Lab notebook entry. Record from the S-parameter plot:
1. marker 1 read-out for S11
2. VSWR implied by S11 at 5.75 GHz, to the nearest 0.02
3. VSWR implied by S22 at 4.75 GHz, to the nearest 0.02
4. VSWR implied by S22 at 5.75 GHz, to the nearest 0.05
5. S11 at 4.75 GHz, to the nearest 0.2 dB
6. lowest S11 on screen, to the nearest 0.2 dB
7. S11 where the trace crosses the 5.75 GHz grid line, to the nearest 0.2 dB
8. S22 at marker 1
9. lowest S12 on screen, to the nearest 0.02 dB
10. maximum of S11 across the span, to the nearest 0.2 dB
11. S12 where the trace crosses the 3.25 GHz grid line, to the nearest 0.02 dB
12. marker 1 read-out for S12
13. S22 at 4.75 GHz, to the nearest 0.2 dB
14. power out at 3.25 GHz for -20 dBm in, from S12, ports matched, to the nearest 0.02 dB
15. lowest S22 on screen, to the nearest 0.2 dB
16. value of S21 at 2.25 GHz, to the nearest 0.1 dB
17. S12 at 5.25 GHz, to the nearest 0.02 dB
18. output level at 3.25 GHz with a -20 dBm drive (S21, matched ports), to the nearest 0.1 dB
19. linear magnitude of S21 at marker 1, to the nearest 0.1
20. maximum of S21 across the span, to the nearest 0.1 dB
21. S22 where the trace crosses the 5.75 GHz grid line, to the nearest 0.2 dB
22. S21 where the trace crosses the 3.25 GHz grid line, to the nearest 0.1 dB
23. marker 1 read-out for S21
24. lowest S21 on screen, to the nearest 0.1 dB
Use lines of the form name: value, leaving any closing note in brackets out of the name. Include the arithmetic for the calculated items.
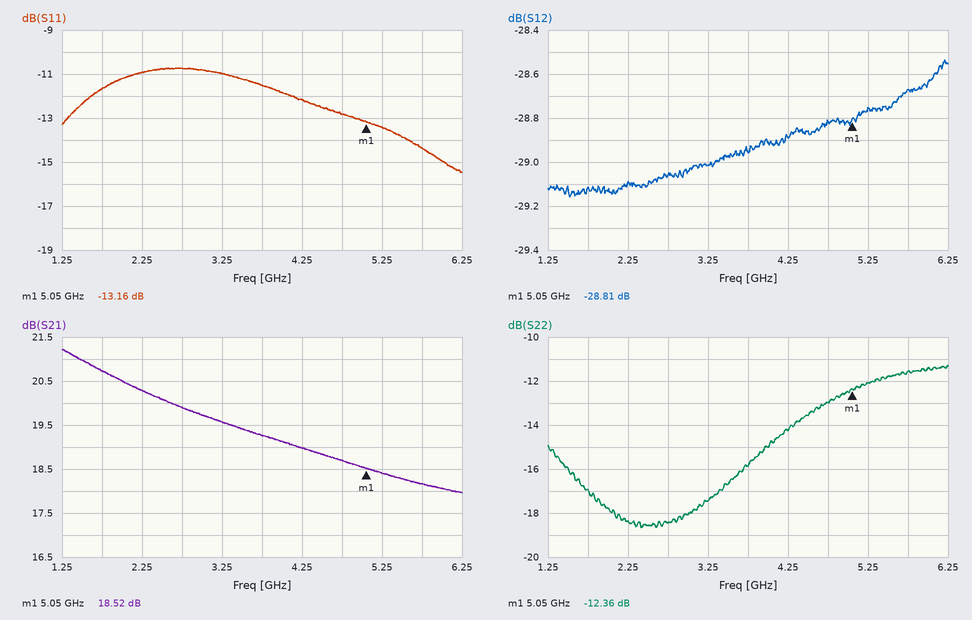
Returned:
marker 1 read-out for S11: -13.16 dB
VSWR implied by S11 at 5.75 GHz, to the nearest 0.02: |Γ| = 10^(-14.4/20) = 0.1905; VSWR = (1 + 0.1905)/(1 − 0.1905) ≈ 1.47, so 1.48 to the nearest 0.02
VSWR implied by S22 at 4.75 GHz, to the nearest 0.02: |Γ| = 10^(-13/20) = 0.2239; VSWR = (1 + 0.2239)/(1 − 0.2239) ≈ 1.58
VSWR implied by S22 at 5.75 GHz, to the nearest 0.05: |Γ| = 10^(-11.6/20) = 0.2630; VSWR = (1 + 0.2630)/(1 − 0.2630) ≈ 1.71, so 1.70 to the nearest 0.05
S11 at 4.75 GHz, to the nearest 0.2 dB: -12.8 dB
lowest S11 on screen, to the nearest 0.2 dB: -15.4 dB
S11 where the trace crosses the 5.75 GHz grid line, to the nearest 0.2 dB: -14.4 dB
S22 at marker 1: -12.36 dB
lowest S12 on screen, to the nearest 0.02 dB: -29.16 dB
maximum of S11 across the span, to the nearest 0.2 dB: -10.8 dB
S12 where the trace crosses the 3.25 GHz grid line, to the nearest 0.02 dB: -29.02 dB
marker 1 read-out for S12: -28.81 dB
S22 at 4.75 GHz, to the nearest 0.2 dB: -13.0 dB
power out at 3.25 GHz for -20 dBm in, from S12, ports matched, to the nearest 0.02 dB: -20 dBm + (-29.02 dB) = -49.02 dBm
lowest S22 on screen, to the nearest 0.2 dB: -18.6 dB
value of S21 at 2.25 GHz, to the nearest 0.1 dB: 20.3 dB
S12 at 5.25 GHz, to the nearest 0.02 dB: -28.76 dB
output level at 3.25 GHz with a -20 dBm drive (S21, matched ports), to the nearest 0.1 dB: -20 dBm + (19.6 dB) = -0.4 dBm
linear magnitude of S21 at marker 1, to the nearest 0.1: 10^(18.52/20) ≈ 8.4
maximum of S21 across the span, to the nearest 0.1 dB: 21.2 dB
S22 where the trace crosses the 5.75 GHz grid line, to the nearest 0.2 dB: -11.6 dB
S21 where the trace crosses the 3.25 GHz grid line, to the nearest 0.1 dB: 19.6 dB
marker 1 read-out for S21: 18.52 dB
lowest S21 on screen, to the nearest 0.1 dB: 18.0 dB
